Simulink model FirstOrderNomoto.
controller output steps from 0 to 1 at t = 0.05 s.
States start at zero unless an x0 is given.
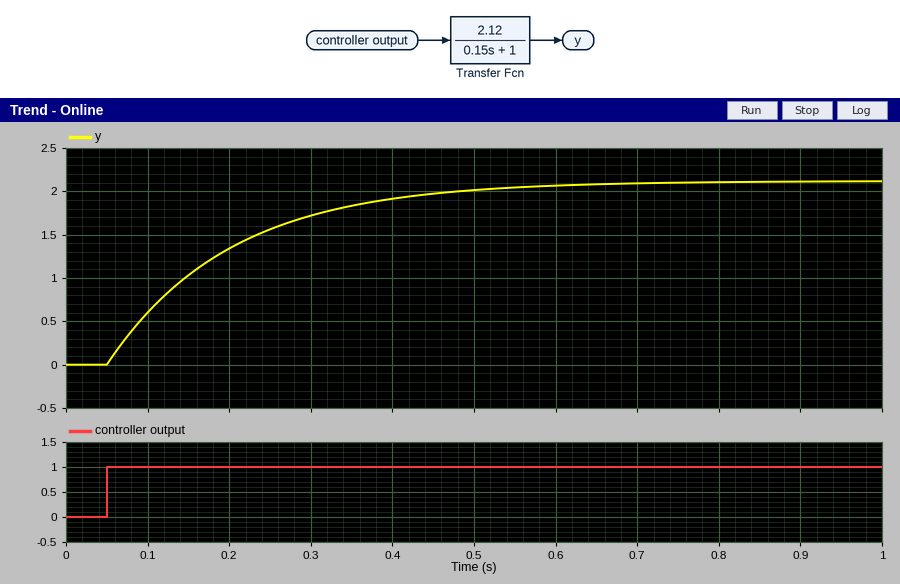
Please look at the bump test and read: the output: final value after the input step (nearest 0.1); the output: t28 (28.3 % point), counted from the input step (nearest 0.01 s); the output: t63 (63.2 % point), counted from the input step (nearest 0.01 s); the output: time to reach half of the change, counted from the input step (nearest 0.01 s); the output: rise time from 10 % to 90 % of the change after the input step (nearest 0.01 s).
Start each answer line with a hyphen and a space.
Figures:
- 2.1
- 0.05 s
- 0.15 s
- 0.10 s
- 0.33 s
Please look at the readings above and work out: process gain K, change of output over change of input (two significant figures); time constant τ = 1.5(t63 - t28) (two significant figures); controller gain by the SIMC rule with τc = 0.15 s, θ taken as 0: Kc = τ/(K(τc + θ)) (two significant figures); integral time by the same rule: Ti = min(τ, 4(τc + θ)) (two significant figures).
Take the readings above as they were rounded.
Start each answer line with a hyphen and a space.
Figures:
- 2.1
- 0.15 s
- 0.48
- 0.15 s
